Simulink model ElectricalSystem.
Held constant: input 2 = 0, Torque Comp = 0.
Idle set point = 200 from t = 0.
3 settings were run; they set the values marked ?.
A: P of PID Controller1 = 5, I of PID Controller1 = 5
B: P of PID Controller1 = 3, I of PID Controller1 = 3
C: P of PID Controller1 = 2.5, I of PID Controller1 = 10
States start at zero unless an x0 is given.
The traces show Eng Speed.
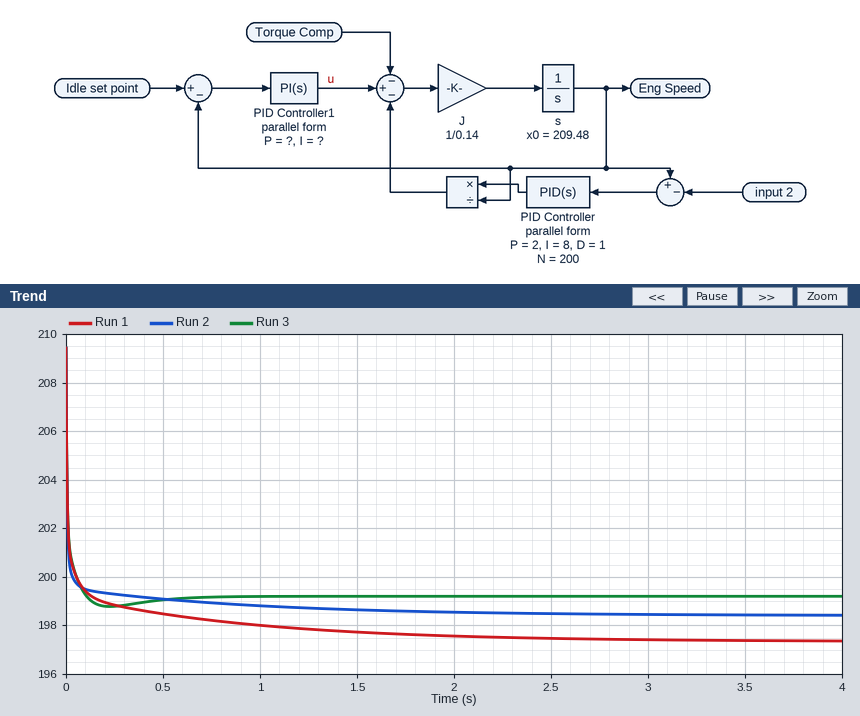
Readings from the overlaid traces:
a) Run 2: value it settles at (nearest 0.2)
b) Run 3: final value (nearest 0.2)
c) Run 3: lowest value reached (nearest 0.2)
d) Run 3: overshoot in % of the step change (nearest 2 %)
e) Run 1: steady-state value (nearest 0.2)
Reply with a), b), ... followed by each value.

a) 198.4
b) 199.2
c) 198.8
d) 4 %
e) 197.4
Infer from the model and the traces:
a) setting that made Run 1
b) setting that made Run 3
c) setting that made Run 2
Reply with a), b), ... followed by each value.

a) B
b) C
c) A
